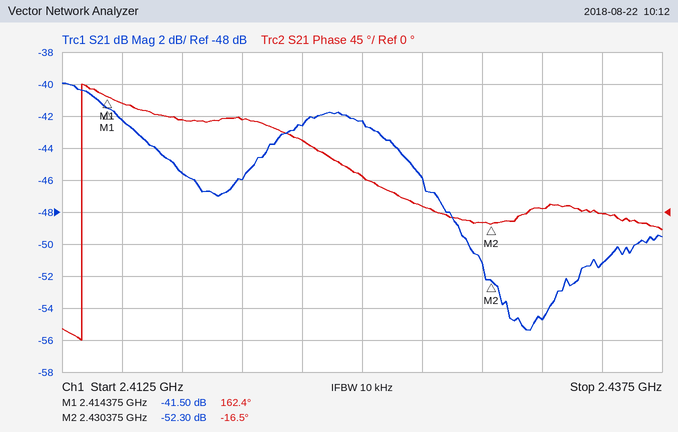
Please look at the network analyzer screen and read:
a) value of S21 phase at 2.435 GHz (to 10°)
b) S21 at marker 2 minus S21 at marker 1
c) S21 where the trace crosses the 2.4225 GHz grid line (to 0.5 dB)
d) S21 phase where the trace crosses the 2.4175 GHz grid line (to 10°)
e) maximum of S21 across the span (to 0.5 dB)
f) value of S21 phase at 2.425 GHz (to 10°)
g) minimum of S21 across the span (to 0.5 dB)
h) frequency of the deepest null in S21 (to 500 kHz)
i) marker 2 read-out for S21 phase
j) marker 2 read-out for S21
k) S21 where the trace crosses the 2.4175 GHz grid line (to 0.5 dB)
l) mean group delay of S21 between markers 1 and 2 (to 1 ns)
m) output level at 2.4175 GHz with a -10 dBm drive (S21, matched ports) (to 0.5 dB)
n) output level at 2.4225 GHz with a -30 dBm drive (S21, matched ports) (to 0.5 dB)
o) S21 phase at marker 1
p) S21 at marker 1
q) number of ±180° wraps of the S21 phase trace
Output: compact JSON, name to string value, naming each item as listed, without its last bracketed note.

{"value of S21 phase at 2.435 GHz": "0°", "S21 at marker 2 minus S21 at marker 1": "-10.80 dB", "S21 where the trace crosses the 2.4225 GHz grid line": "-42.5 dB", "S21 phase where the trace crosses the 2.4175 GHz grid line": "130°", "maximum of S21 across the span": "-40.0 dB", "value of S21 phase at 2.425 GHz": "50°", "minimum of S21 across the span": "-55.5 dB", "frequency of the deepest null in S21": "2.4320 GHz", "marker 2 read-out for S21 phase": "-16.5°", "marker 2 read-out for S21": "-52.30 dB", "S21 where the trace crosses the 2.4175 GHz grid line": "-45.5 dB", "mean group delay of S21 between markers 1 and 2": "31 ns", "output level at 2.4175 GHz with a -10 dBm drive (S21, matched ports)": "-55.5 dBm", "output level at 2.4225 GHz with a -30 dBm drive (S21, matched ports)": "-72.5 dBm", "S21 phase at marker 1": "162.4°", "S21 at marker 1": "-41.50 dB", "number of ±180° wraps of the S21 phase trace": "1"}
